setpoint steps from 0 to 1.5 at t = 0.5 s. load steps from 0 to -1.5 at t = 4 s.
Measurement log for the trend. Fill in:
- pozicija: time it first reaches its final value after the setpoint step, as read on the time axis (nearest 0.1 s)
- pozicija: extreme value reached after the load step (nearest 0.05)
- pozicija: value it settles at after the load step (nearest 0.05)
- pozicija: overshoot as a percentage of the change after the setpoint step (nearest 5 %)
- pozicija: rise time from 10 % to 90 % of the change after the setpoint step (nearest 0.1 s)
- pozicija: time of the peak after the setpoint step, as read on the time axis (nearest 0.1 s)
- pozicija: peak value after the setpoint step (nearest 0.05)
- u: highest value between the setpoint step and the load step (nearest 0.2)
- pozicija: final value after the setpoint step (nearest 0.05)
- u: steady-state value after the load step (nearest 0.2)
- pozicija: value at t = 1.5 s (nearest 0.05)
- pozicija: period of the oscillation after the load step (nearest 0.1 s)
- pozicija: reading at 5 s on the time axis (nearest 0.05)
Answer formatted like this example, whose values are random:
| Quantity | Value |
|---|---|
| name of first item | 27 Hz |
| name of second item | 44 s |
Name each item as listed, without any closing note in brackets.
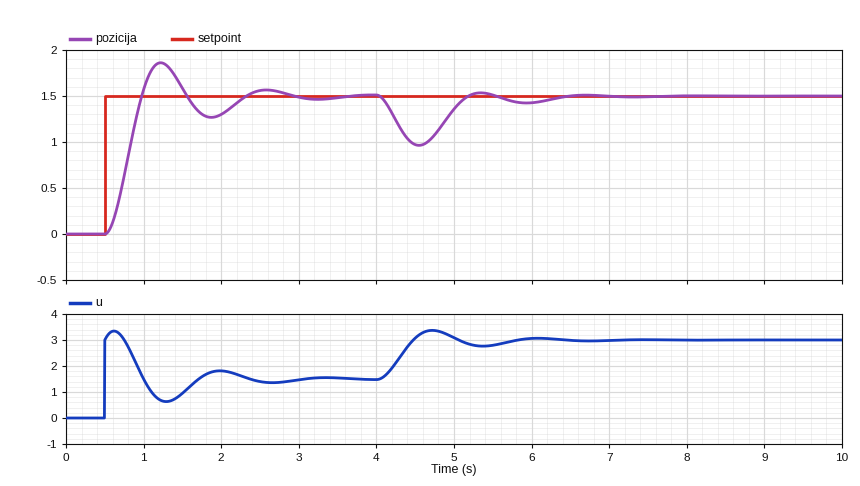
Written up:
| Quantity | Value |
|---|---|
| pozicija: time it first reaches its final value after the setpoint step, as read on the time axis | 1.0 s |
| pozicija: extreme value reached after the load step | 0.95 |
| pozicija: value it settles at after the load step | 1.50 |
| pozicija: overshoot as a percentage of the change after the setpoint step | 25 % |
| pozicija: rise time from 10 % to 90 % of the change after the setpoint step | 0.3 s |
| pozicija: time of the peak after the setpoint step, as read on the time axis | 1.2 s |
| pozicija: peak value after the setpoint step | 1.85 |
| u: highest value between the setpoint step and the load step | 3.4 |
| pozicija: final value after the setpoint step | 1.50 |
| u: steady-state value after the load step | 3.0 |
| pozicija: value at t = 1.5 s | 1.60 |
| pozicija: period of the oscillation after the load step | 1.4 s |
| pozicija: reading at 5 s on the time axis | 1.35 |
